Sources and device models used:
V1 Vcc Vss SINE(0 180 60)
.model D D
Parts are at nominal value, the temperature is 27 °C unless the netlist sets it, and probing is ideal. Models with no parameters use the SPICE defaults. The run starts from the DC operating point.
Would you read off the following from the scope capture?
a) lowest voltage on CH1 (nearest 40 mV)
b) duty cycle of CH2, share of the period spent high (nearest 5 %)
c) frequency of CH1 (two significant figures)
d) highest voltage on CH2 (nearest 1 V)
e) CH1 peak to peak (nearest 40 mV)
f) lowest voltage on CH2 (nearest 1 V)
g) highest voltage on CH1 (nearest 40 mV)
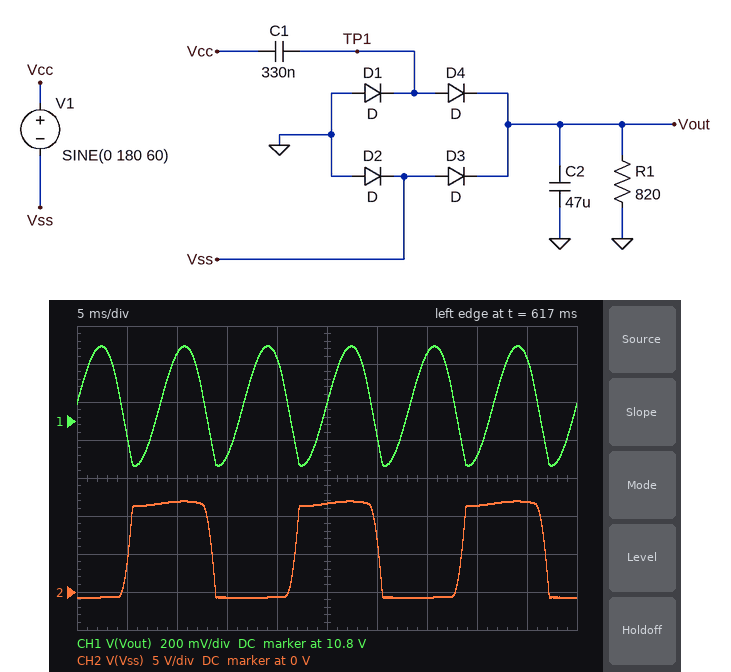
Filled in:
10.56 V
50 %
120 Hz
12 V
640 mV
-1 V
11.20 V
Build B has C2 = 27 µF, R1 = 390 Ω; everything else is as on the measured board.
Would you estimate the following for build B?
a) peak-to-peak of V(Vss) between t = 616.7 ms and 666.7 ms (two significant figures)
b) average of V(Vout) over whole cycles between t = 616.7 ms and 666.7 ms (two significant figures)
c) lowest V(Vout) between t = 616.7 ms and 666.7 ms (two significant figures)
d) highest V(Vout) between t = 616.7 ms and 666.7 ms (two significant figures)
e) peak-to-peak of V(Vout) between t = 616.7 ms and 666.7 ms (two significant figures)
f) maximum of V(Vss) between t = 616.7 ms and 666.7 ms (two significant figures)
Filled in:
7.3 V
5.4 V
4.8 V
5.8 V
1.0 V
6.6 V
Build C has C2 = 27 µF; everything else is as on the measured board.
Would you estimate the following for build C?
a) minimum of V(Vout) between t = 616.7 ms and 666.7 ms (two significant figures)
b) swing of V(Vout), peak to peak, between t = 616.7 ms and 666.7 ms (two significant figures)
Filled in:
10 V
1.1 V
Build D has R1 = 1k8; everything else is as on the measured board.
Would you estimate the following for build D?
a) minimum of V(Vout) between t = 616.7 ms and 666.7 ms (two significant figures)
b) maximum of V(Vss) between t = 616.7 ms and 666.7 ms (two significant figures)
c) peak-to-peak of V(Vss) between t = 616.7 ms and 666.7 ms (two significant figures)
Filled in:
22 V
23 V
24 V
